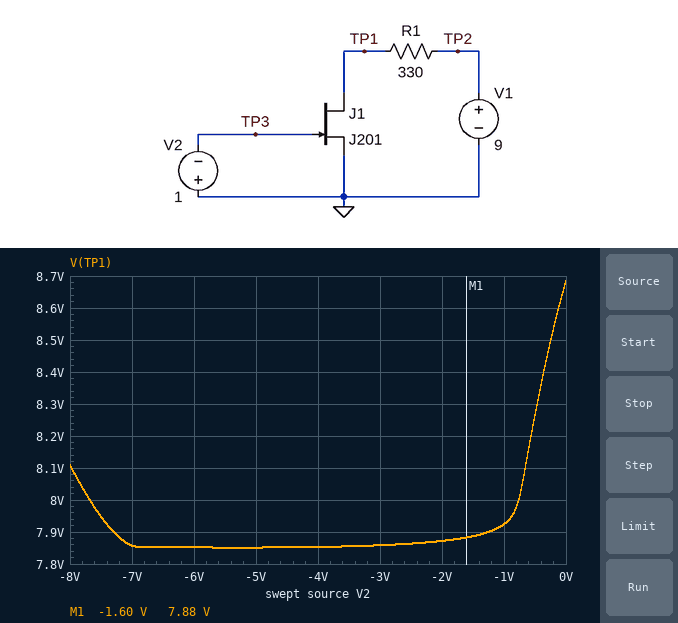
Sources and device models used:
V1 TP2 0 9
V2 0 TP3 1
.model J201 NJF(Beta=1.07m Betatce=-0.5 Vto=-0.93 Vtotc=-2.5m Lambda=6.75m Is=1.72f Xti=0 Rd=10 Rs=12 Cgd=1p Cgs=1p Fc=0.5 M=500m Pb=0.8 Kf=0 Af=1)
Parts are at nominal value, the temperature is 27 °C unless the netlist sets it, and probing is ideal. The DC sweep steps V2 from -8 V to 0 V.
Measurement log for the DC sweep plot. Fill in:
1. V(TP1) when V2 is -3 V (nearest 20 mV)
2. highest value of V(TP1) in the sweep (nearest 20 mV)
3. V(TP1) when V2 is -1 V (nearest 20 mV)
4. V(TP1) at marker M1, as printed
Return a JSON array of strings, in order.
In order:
["7.86 V", "8.68 V", "7.92 V", "7.88 V"]
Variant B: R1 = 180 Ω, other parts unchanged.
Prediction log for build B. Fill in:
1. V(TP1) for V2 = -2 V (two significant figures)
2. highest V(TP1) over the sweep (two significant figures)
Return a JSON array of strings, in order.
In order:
["8.4 V", "8.8 V"]
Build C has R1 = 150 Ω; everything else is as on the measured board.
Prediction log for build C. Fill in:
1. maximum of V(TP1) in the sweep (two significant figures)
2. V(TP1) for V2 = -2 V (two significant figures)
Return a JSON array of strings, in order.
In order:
["8.9 V", "8.5 V"]
